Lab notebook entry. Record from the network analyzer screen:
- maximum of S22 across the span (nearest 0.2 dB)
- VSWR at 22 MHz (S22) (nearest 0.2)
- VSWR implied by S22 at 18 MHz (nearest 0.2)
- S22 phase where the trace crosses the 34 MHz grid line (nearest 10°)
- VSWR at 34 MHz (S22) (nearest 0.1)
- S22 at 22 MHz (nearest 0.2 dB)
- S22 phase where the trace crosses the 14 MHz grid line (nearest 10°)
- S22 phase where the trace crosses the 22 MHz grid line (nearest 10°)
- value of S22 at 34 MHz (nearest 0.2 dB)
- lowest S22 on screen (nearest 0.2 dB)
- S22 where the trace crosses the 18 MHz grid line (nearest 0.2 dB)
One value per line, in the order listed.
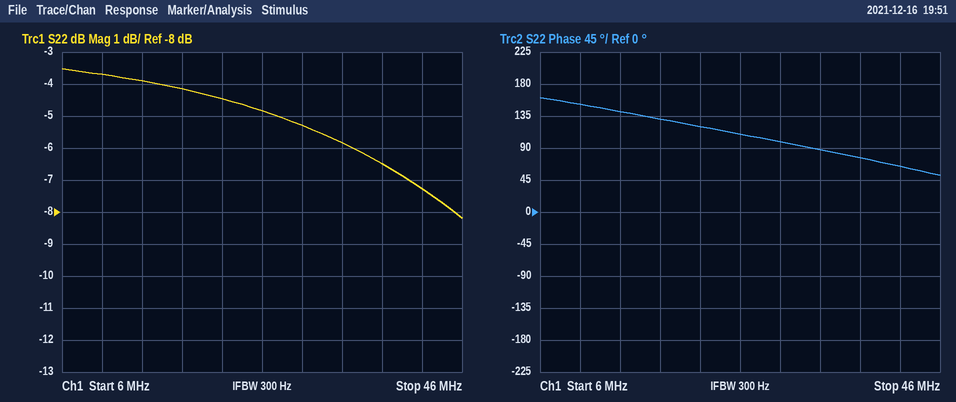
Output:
-3.6 dB
4.0
4.2
90°
3.1
-4.4 dB
140°
120°
-5.8 dB
-8.2 dB
-4.2 dB
